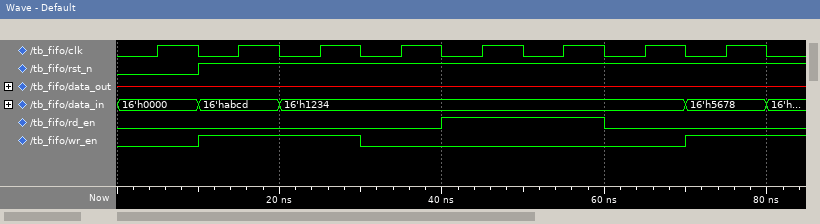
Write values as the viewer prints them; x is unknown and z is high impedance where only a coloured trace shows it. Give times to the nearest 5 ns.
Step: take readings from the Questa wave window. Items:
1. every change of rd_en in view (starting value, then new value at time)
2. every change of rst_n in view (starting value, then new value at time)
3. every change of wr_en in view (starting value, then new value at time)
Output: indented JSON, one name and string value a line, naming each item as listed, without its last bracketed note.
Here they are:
{
  "every change of rd_en in view": "0, 1 at 40 ns, 0 at 60 ns",
  "every change of rst_n in view": "0, 1 at 10 ns",
  "every change of wr_en in view": "0, 1 at 10 ns, 0 at 30 ns, 1 at 70 ns"
}
